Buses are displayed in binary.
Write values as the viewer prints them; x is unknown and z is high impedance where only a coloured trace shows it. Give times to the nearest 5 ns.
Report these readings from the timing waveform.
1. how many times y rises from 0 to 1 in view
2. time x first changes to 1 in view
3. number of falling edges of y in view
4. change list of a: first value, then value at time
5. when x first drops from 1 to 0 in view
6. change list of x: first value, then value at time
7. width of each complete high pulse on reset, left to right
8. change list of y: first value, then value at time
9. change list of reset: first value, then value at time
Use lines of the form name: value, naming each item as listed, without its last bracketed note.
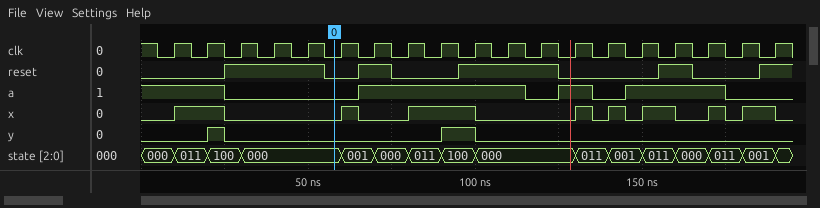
how many times y rises from 0 to 1 in view: 2
time x first changes to 1 in view: 10 ns
number of falling edges of y in view: 2
change list of a: first value, then value at time: 1, 0 at 25 ns, 1 at 65 ns, 0 at 115 ns, 1 at 125 ns, 0 at 135 ns, 1 at 145 ns, 0 at 175 ns
when x first drops from 1 to 0 in view: 25 ns
change list of x: first value, then value at time: 0, 1 at 10 ns, 0 at 25 ns, 1 at 60 ns, 0 at 65 ns, 1 at 80 ns, 0 at 100 ns, 1 at 130 ns, 0 at 135 ns, 1 at 140 ns, 0 at 145 ns, 1 at 150 ns, 0 at 160 ns, 1 at 170 ns, 0 at 175 ns, 1 at 180 ns, 0 at 190 ns
width of each complete high pulse on reset, left to right: 30 ns, 10 ns, 30 ns, 10 ns
change list of y: first value, then value at time: 0, 1 at 20 ns, 0 at 25 ns, 1 at 90 ns, 0 at 100 ns
change list of reset: first value, then value at time: 0, 1 at 25 ns, 0 at 55 ns, 1 at 65 ns, 0 at 75 ns, 1 at 95 ns, 0 at 125 ns, 1 at 155 ns, 0 at 165 ns, 1 at 185 ns
